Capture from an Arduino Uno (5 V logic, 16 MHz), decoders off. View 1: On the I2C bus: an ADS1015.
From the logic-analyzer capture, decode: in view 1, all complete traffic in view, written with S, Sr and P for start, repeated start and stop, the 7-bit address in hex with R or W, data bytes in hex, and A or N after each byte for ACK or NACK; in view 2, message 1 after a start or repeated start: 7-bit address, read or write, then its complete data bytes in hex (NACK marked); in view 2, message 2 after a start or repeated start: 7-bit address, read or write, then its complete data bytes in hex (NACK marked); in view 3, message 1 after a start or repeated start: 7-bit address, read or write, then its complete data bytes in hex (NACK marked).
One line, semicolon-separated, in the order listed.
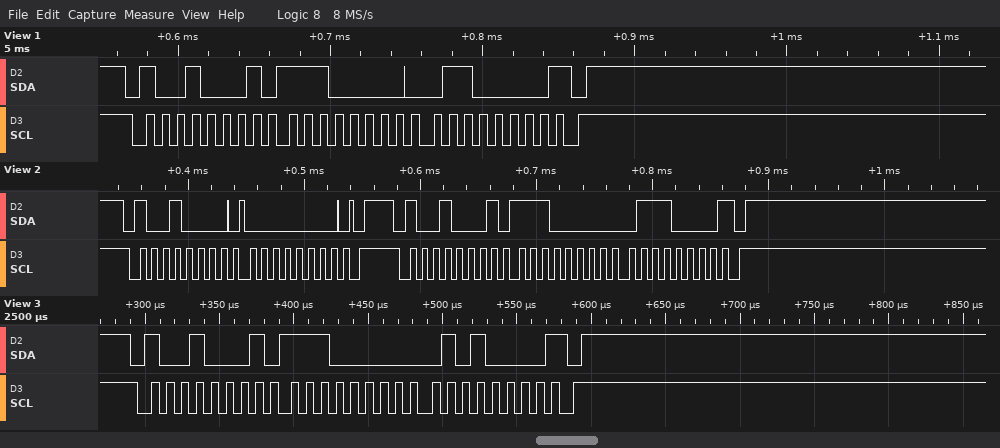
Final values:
S 48R A E0 A 60 N P; 0x48 write: 00; 0x48 read: E0 70 NACK; 0x48 read: E0 50 NACK
